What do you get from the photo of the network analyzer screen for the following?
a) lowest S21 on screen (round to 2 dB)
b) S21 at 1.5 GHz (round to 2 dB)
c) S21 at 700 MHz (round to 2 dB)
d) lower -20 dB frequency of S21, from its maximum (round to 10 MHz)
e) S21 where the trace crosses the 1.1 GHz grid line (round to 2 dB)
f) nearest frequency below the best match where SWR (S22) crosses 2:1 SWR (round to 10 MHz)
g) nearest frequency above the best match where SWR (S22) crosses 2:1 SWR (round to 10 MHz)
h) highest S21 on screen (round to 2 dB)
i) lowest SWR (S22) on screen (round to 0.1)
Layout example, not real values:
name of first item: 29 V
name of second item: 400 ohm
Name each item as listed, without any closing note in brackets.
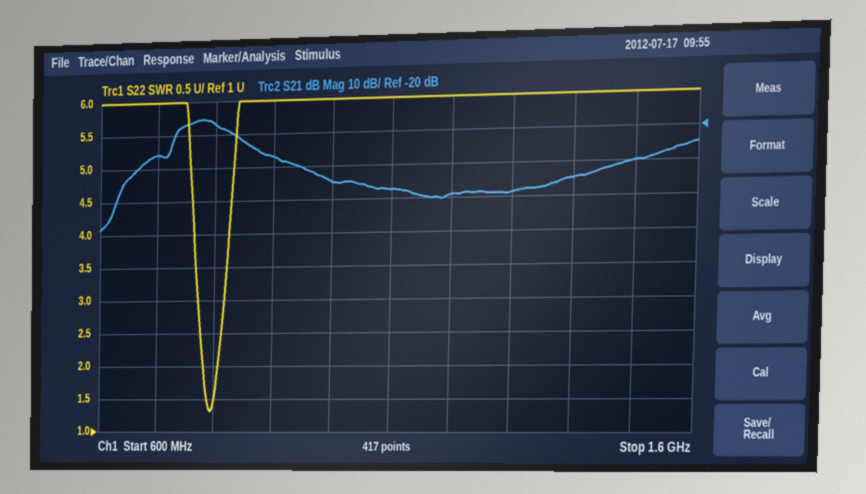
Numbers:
lowest S21 on screen: -48 dB
S21 at 1.5 GHz: -30 dB
S21 at 700 MHz: -26 dB
lower -20 dB frequency of S21, from its maximum: 640 MHz
S21 where the trace crosses the 1.1 GHz grid line: -38 dB
nearest frequency below the best match where SWR (S22) crosses 2:1 SWR: 780 MHz
nearest frequency above the best match where SWR (S22) crosses 2:1 SWR: 810 MHz
highest S21 on screen: -16 dB
lowest SWR (S22) on screen: 1.3
